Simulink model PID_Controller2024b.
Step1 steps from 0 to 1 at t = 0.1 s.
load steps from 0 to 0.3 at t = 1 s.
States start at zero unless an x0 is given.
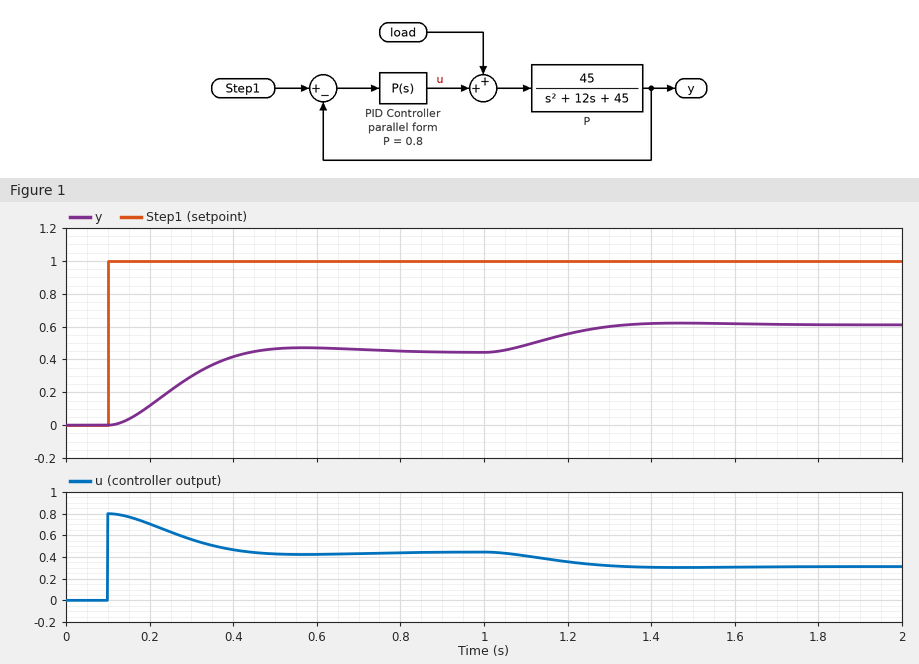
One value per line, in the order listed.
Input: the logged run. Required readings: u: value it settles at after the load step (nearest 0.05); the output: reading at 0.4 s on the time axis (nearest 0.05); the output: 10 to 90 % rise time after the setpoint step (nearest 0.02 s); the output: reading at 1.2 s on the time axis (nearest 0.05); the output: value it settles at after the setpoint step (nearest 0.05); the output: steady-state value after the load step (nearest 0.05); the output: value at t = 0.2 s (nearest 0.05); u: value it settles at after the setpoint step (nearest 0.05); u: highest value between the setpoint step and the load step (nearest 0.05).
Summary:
0.30
0.40
0.22 s
0.55
0.45
0.60
0.10
0.45
0.80
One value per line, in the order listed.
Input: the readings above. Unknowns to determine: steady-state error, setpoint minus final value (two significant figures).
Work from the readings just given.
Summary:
0.55
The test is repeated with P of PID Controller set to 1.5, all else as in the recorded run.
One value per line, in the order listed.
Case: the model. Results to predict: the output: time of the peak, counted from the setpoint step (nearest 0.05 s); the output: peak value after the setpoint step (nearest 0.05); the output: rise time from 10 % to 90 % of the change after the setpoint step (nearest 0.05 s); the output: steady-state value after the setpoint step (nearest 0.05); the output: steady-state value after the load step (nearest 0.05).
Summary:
0.35 s
0.65
0.15 s
0.60
0.70
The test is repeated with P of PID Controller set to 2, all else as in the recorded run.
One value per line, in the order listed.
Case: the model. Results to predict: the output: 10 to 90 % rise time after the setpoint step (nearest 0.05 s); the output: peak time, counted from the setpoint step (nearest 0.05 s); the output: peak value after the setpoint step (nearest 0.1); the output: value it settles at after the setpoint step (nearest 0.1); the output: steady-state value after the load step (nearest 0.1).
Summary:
0.15 s
0.30 s
0.8
0.7
0.8
